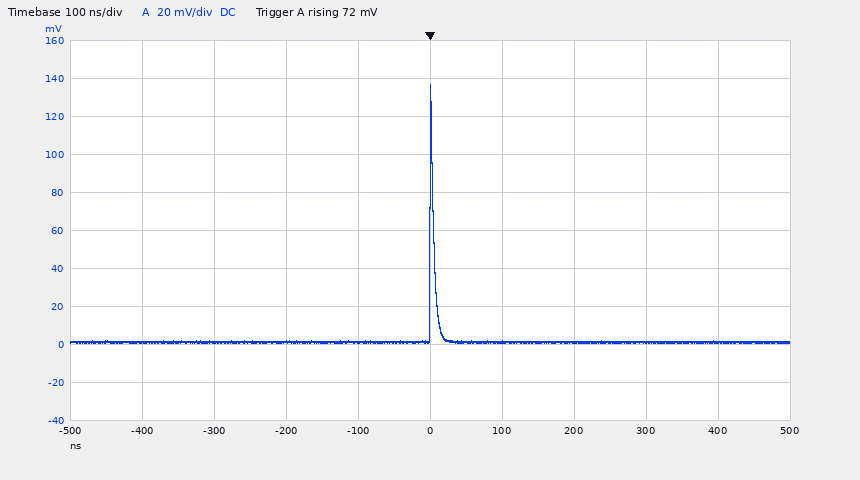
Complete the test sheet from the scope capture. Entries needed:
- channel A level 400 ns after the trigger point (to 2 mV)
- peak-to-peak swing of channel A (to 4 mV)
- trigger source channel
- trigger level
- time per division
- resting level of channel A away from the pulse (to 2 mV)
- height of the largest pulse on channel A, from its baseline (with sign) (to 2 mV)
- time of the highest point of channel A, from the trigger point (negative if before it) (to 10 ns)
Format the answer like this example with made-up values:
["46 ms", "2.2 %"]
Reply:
["2 mV", "136 mV", "channel A", "72 mV", "100 ns", "2 mV", "+136 mV", "0 ns"]
